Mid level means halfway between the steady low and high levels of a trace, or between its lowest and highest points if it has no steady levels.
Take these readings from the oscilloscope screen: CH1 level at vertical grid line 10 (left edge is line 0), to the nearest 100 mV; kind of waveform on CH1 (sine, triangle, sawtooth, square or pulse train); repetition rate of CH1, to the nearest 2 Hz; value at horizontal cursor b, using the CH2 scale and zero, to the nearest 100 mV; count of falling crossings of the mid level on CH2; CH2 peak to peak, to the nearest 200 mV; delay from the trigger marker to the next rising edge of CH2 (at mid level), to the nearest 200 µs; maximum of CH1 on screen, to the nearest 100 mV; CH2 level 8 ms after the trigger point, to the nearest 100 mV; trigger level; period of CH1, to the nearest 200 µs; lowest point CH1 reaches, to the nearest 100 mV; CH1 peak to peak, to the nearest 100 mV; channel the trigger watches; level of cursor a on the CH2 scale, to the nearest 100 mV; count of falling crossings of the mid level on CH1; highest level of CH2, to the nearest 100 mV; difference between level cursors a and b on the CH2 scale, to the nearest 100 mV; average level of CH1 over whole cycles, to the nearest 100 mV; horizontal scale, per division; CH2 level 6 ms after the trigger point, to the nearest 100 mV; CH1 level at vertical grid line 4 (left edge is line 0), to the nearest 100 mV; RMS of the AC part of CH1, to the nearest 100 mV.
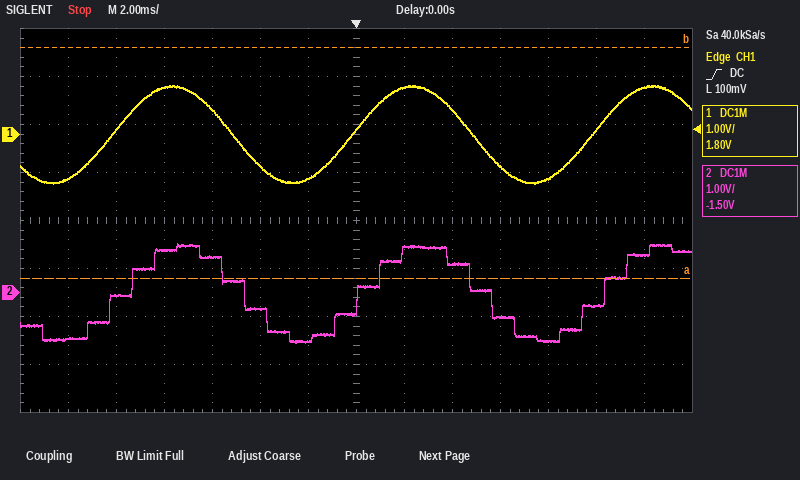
-700 mV
sine
100 Hz
5.1 V
2
2.0 V
10.4 ms
1.0 V
-1.0 V
100 mV
10.0 ms
-1.0 V
2.0 V
CH1
300 mV
2
1.0 V
4.8 V
0.0 V
2 ms
-500 mV
500 mV
700 mV
